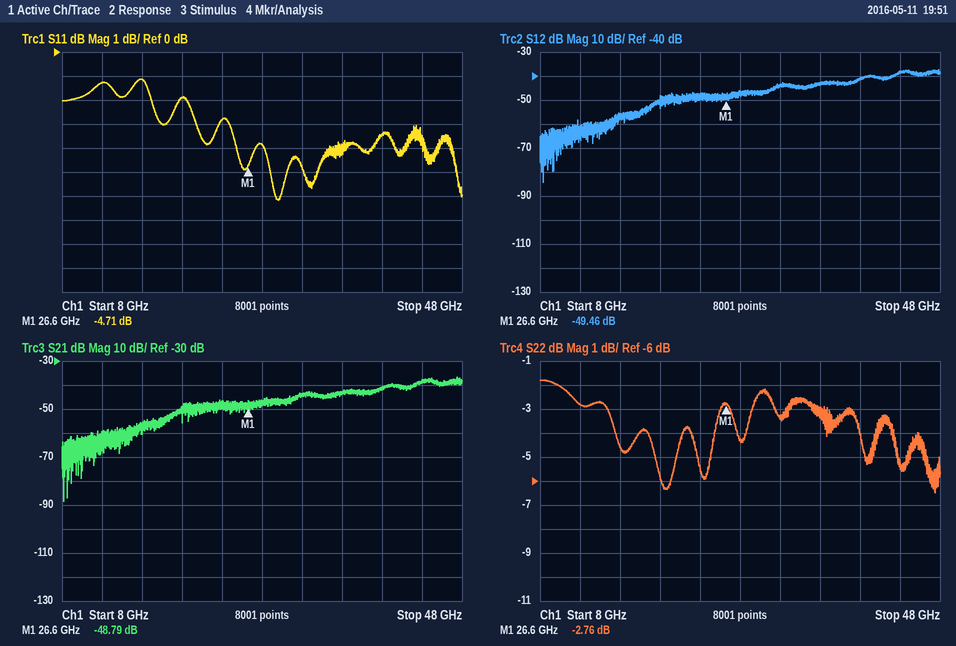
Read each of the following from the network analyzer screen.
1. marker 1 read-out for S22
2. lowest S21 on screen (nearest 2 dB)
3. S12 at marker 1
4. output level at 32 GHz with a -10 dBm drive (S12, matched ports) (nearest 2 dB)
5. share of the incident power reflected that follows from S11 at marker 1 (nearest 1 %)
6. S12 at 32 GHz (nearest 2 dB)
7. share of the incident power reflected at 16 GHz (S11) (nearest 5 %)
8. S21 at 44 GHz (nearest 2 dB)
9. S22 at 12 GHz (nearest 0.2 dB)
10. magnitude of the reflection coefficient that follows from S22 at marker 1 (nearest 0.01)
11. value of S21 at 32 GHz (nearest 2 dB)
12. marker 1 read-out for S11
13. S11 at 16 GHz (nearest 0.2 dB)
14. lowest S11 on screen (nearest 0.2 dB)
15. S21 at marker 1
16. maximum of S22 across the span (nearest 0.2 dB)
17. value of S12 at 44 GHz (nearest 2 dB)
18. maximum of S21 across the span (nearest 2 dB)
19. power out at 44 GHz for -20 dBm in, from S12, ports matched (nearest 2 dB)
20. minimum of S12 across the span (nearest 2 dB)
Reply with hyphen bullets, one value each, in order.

- -2.76 dB
- -88 dB
- -49.46 dB
- -54 dBm
- 34 %
- -44 dB
- 75 %
- -38 dB
- -2.8 dB
- 0.73
- -44 dB
- -4.71 dB
- -1.2 dB
- -6.2 dB
- -48.79 dB
- -1.8 dB
- -38 dB
- -36 dB
- -58 dBm
- -84 dB
